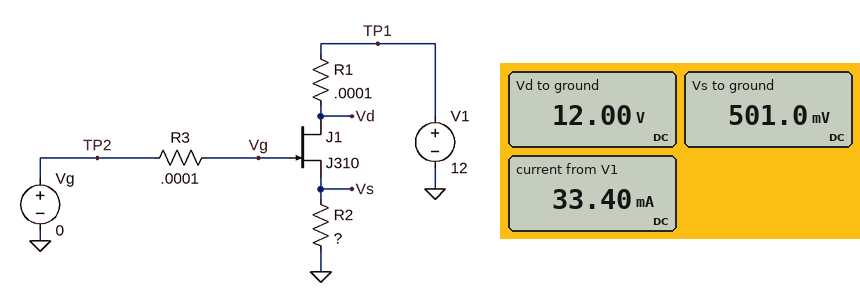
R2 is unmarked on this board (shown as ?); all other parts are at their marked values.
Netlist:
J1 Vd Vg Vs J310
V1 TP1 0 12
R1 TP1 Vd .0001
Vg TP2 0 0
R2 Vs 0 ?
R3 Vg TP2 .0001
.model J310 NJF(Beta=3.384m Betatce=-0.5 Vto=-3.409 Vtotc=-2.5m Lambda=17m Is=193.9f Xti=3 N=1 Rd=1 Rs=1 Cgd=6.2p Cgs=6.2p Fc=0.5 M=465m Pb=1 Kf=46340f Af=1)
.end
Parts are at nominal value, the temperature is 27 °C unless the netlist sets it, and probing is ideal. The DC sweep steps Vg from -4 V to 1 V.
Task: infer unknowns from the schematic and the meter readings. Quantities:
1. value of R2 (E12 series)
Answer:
15 Ω
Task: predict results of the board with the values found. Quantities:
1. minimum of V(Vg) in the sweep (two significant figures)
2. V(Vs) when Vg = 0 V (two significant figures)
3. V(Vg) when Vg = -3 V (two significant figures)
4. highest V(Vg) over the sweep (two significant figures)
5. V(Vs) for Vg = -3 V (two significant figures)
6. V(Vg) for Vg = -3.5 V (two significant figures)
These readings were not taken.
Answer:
-4.0 V
500 mV
-3.0 V
1.0 V
9.7 mV
-3.5 V
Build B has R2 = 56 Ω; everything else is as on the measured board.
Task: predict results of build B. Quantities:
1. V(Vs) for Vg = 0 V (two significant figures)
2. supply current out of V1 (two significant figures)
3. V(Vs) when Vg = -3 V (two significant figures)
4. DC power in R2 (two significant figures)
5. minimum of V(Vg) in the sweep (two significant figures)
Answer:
1.1 V
20 mA
32 mV
23 mW
-4.0 V
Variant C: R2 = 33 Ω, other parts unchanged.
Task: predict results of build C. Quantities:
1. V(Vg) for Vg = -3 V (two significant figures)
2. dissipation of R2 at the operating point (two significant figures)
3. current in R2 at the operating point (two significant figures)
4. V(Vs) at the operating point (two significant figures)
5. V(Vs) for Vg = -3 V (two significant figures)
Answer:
-3.0 V
22 mW
26 mA
850 mV
20 mV
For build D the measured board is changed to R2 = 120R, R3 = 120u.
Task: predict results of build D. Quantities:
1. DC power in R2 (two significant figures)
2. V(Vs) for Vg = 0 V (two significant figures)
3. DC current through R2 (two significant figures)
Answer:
21 mW
1.6 V
13 mA
